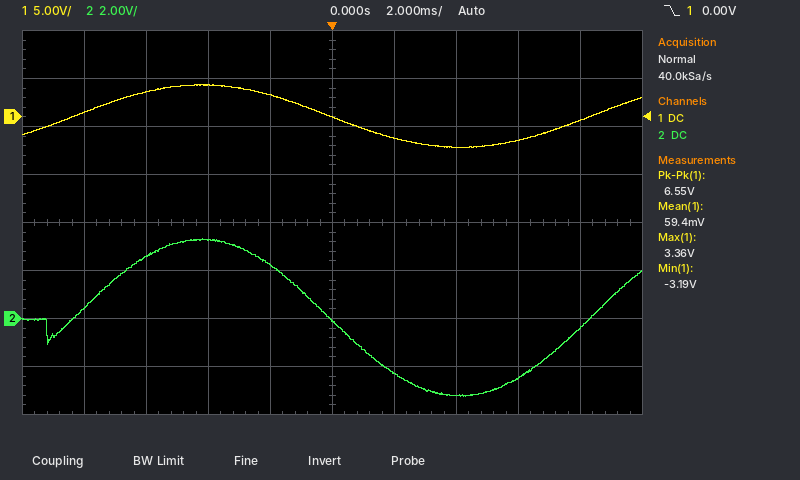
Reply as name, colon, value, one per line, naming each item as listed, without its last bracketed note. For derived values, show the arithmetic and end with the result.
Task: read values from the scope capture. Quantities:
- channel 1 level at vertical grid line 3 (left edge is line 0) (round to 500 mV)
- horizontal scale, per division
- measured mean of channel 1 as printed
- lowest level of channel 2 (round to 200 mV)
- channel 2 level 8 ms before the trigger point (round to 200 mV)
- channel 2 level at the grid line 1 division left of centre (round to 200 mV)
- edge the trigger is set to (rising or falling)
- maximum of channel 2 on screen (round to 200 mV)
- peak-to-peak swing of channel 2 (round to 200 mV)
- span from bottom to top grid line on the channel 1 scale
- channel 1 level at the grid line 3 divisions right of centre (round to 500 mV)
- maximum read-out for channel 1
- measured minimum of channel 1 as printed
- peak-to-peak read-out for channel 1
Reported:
channel 1 level at vertical grid line 3 (left edge is line 0): 3.5 V
horizontal scale, per division: 2 ms
measured mean of channel 1 as printed: 59.4 mV
lowest level of channel 2: -3.2 V
channel 2 level 8 ms before the trigger point: 400 mV
channel 2 level at the grid line 1 division left of centre: 2.2 V
edge the trigger is set to: falling
maximum of channel 2 on screen: 3.4 V
peak-to-peak swing of channel 2: 3.4 V − (-3.2 V) = 6.6 V
span from bottom to top grid line on the channel 1 scale: 40 V
channel 1 level at the grid line 3 divisions right of centre: -2.5 V
maximum read-out for channel 1: 3.36 V
measured minimum of channel 1 as printed: -3.19 V
peak-to-peak read-out for channel 1: 6.55 V
